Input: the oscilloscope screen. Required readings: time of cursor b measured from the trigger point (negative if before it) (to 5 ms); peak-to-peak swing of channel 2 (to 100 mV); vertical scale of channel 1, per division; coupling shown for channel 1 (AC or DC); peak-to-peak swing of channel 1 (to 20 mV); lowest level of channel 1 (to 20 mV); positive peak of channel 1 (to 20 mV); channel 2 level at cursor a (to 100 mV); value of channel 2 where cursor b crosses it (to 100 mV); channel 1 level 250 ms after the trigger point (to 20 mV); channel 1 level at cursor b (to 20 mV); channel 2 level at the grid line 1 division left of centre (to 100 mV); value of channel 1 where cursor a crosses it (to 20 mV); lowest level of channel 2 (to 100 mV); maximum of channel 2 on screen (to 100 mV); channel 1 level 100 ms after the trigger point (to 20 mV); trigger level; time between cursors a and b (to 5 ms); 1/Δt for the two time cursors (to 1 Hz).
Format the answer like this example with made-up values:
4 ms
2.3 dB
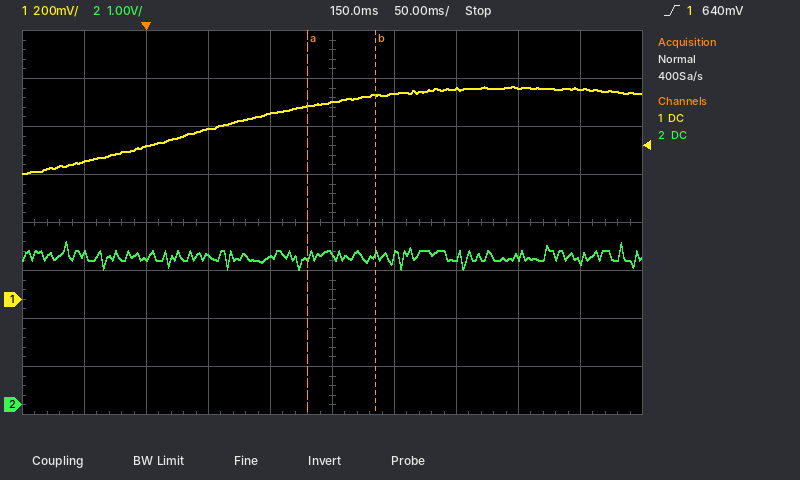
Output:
+185 ms
600 mV
200 mV
DC
360 mV
520 mV
880 mV
3.1 V
3.1 V
880 mV
860 mV
3.1 V
800 mV
2.8 V
3.4 V
780 mV
640 mV
55 ms
18 Hz
